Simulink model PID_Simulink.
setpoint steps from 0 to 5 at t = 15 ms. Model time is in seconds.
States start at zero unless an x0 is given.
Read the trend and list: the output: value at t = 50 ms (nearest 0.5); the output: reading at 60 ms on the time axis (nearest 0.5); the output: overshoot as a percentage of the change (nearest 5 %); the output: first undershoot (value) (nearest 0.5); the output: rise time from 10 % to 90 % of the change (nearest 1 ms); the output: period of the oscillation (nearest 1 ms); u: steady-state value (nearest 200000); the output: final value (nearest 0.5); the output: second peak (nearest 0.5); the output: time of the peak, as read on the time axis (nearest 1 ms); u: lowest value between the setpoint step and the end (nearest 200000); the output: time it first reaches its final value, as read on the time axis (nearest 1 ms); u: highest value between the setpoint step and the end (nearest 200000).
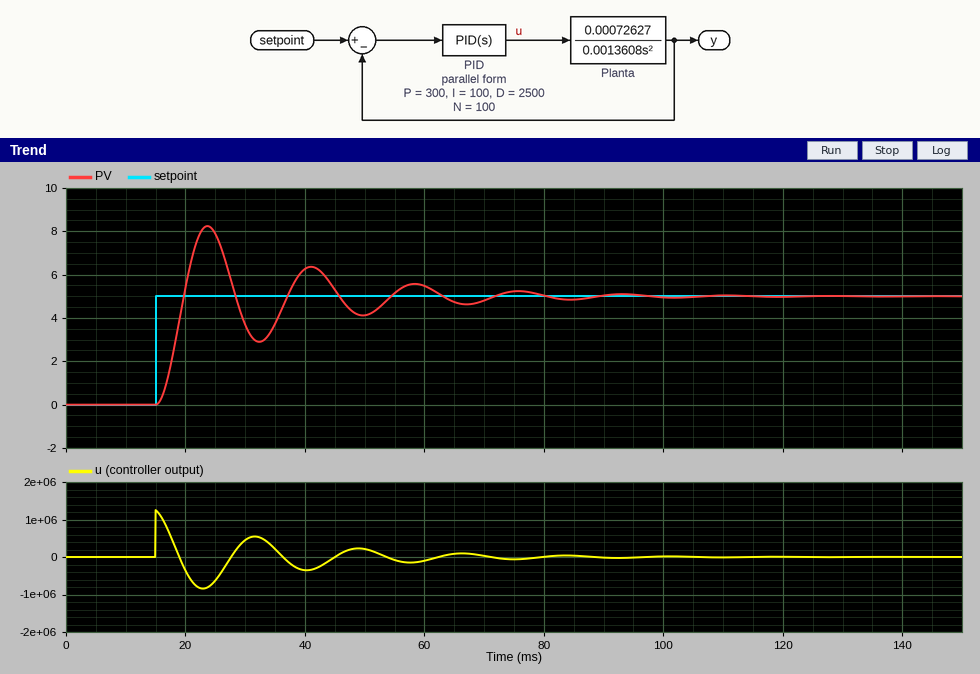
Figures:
4.0
5.5
65 %
3.0
3 ms
17 ms
0
5.0
6.5
24 ms
-800000
20 ms
1200000
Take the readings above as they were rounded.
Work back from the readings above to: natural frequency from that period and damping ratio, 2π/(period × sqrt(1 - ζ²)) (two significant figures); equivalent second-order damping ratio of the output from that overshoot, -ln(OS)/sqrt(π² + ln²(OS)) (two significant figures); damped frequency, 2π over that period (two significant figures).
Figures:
0.37 rad/ms
0.14
0.37 rad/ms
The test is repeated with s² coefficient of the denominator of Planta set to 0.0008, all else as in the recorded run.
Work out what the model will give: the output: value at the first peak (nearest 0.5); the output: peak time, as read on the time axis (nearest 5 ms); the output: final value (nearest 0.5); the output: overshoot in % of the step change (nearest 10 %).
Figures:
8.5
20 ms
5.0
70 %
